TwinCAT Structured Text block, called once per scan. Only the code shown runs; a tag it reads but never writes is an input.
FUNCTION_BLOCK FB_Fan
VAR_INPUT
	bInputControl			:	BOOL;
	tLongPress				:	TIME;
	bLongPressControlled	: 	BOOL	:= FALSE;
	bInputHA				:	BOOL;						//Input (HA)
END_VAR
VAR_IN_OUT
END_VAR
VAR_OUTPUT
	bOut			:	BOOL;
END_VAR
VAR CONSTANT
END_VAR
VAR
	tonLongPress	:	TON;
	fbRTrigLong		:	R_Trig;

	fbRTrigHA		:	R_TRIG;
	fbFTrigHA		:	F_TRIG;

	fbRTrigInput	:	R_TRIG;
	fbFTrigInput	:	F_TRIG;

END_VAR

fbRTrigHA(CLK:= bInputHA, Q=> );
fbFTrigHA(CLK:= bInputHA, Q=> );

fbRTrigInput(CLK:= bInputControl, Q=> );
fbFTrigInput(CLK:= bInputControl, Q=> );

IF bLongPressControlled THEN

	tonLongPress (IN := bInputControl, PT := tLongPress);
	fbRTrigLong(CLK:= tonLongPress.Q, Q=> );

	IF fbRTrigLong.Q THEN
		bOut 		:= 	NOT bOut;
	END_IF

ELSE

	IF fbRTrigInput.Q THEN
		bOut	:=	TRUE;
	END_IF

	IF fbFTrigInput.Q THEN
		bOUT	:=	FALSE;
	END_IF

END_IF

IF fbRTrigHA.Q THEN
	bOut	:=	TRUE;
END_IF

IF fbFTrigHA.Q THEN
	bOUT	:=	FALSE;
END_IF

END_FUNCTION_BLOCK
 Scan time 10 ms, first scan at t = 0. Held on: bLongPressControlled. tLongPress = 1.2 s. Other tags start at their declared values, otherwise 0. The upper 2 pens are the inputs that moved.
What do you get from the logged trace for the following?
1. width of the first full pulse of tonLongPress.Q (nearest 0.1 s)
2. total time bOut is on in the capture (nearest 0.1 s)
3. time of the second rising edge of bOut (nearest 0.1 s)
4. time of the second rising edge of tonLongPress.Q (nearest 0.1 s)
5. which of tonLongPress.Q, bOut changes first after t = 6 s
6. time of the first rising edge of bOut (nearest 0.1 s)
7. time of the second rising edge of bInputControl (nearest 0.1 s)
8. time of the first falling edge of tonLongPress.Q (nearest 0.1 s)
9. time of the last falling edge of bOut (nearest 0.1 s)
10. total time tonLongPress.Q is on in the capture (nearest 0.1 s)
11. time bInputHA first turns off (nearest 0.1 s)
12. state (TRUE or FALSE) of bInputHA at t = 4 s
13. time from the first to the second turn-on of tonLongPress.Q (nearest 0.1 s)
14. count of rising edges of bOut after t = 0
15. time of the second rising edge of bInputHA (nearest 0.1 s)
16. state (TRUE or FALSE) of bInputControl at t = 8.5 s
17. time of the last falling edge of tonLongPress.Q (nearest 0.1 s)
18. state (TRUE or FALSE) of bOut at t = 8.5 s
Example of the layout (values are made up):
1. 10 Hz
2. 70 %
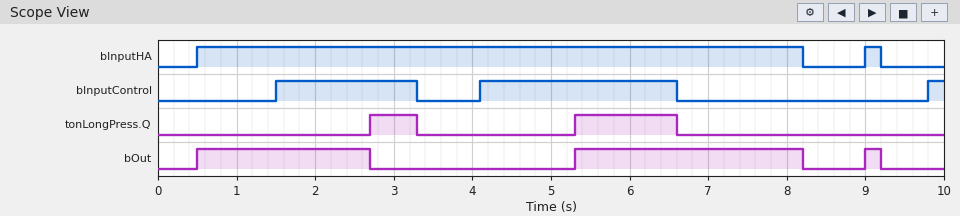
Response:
1. 0.6 s
2. 5.3 s
3. 5.3 s
4. 5.3 s
5. tonLongPress.Q
6. 0.5 s
7. 4.1 s
8. 3.3 s
9. 9.2 s
10. 1.9 s
11. 8.2 s
12. TRUE
13. 2.6 s
14. 3
15. 9.0 s
16. FALSE
17. 6.6 s
18. FALSE
